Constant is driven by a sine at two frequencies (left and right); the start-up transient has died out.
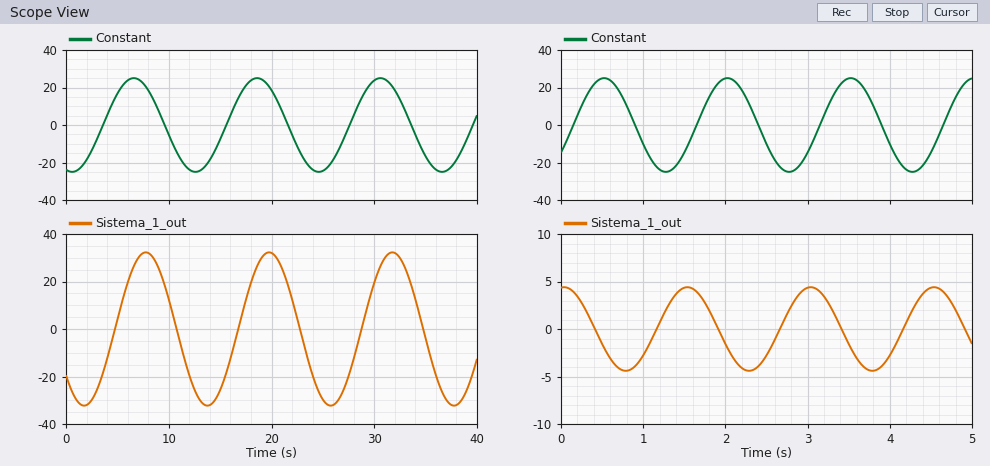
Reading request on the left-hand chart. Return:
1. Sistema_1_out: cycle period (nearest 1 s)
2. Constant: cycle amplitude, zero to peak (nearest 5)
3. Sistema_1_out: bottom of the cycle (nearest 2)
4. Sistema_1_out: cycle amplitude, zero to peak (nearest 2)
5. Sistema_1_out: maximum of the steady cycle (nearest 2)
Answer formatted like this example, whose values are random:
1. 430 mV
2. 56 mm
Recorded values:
1. 12 s
2. 25
3. -32
4. 32
5. 32
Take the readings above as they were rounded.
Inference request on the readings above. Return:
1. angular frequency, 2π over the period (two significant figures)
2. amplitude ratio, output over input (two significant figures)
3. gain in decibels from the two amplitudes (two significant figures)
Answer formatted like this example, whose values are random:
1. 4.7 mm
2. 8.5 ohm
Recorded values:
1. 0.52 rad/s
2. 1.3
3. 2.1 dB
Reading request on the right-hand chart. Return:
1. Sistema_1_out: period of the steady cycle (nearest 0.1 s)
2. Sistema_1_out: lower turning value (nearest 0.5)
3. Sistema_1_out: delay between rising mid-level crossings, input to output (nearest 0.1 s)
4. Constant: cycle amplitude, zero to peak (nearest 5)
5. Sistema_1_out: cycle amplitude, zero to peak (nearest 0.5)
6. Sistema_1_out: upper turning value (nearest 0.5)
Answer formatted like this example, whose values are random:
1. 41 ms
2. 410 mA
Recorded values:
1. 1.5 s
2. -4.5
3. 1.0 s
4. 25
5. 4.5
6. 4.5
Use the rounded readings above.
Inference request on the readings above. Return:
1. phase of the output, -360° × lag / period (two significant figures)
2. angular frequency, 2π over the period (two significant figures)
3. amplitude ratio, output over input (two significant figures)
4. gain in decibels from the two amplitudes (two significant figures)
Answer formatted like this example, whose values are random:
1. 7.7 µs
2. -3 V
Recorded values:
1. -240°
2. 4.2 rad/s
3. 0.18
4. -15 dB
